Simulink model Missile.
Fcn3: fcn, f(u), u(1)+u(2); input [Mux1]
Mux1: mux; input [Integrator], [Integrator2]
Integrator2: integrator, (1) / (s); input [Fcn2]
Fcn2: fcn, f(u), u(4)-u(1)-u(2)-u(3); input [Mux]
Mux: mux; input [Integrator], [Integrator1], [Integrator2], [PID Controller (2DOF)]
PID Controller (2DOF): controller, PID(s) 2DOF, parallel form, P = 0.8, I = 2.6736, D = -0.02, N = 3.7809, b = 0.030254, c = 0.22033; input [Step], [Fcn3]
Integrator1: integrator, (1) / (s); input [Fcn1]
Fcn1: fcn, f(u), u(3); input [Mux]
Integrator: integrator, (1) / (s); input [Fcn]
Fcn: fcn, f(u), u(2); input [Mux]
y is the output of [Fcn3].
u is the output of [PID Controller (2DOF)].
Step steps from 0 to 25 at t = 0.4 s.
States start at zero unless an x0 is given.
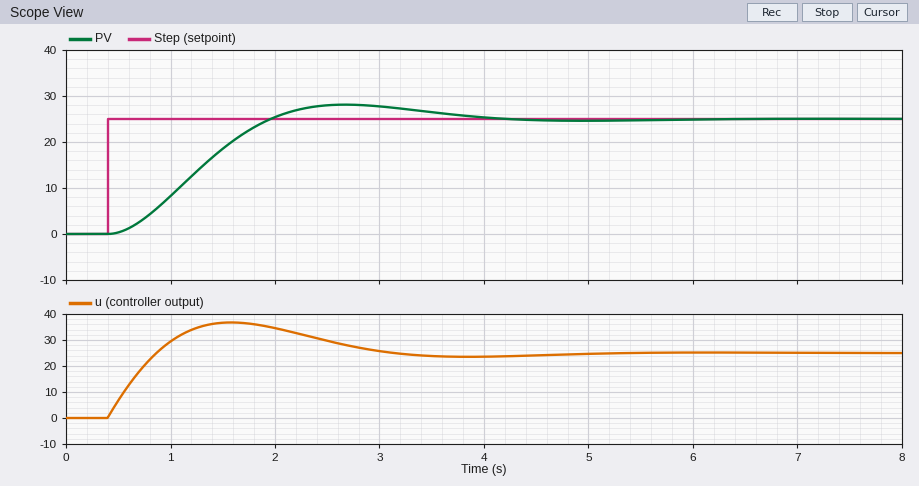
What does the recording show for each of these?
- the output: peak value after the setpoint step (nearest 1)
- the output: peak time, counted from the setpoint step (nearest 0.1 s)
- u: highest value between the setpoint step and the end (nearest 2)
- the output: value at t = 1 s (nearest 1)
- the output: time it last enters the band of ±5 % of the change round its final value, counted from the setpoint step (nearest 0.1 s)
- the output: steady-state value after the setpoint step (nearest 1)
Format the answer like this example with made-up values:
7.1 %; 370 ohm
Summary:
28; 2.3 s; 36; 8; 3.2 s; 25
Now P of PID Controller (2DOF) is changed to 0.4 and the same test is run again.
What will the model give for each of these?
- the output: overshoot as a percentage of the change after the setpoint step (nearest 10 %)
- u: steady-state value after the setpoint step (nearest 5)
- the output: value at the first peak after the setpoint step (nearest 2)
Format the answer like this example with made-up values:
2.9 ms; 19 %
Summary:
20 %; 25; 30
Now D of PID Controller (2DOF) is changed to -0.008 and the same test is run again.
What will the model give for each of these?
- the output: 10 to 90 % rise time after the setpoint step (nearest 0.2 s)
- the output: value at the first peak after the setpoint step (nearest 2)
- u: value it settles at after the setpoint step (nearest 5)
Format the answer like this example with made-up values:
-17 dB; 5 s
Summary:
1.0 s; 28; 25
